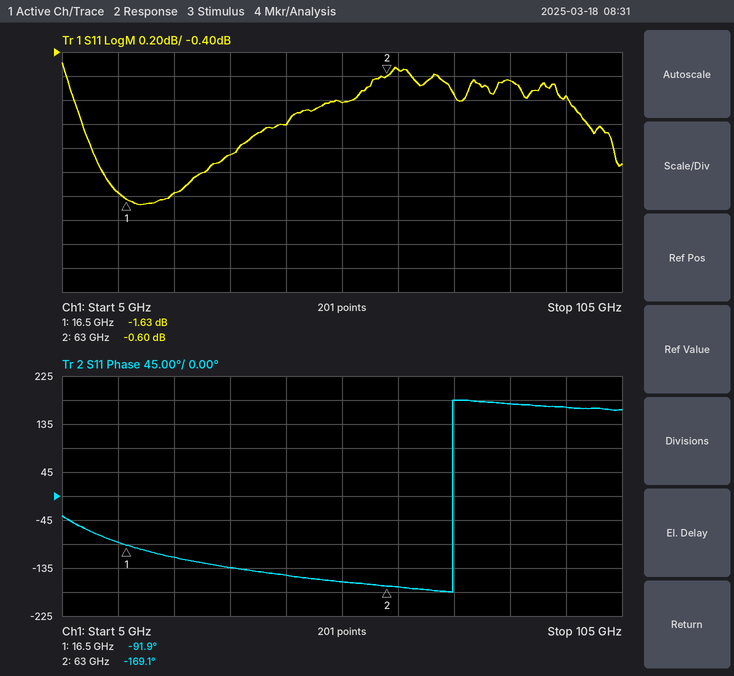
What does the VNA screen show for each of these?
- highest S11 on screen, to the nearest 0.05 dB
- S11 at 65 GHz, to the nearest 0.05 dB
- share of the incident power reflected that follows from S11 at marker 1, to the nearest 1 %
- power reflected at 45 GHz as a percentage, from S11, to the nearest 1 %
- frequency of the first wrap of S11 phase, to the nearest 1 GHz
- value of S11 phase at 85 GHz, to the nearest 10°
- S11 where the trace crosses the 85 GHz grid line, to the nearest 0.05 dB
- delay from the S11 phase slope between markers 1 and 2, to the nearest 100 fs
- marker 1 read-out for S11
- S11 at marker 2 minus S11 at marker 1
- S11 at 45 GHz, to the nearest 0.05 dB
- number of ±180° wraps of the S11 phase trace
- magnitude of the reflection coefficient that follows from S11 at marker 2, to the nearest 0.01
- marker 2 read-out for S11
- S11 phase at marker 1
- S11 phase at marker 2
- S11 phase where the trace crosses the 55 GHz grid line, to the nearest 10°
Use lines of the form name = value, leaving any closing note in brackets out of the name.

highest S11 on screen, to the nearest 0.05 dB = -0.50 dB
S11 at 65 GHz, to the nearest 0.05 dB = -0.55 dB
share of the incident power reflected that follows from S11 at marker 1, to the nearest 1 % = 69 %
power reflected at 45 GHz as a percentage, from S11, to the nearest 1 % = 79 %
frequency of the first wrap of S11 phase, to the nearest 1 GHz = 75 GHz
value of S11 phase at 85 GHz, to the nearest 10° = 170°
S11 where the trace crosses the 85 GHz grid line, to the nearest 0.05 dB = -0.65 dB
delay from the S11 phase slope between markers 1 and 2, to the nearest 100 fs = 4.6 ps
marker 1 read-out for S11 = -1.63 dB
S11 at marker 2 minus S11 at marker 1 = 1.03 dB
S11 at 45 GHz, to the nearest 0.05 dB = -1.00 dB
number of ±180° wraps of the S11 phase trace = 1
magnitude of the reflection coefficient that follows from S11 at marker 2, to the nearest 0.01 = 0.93
marker 2 read-out for S11 = -0.60 dB
S11 phase at marker 1 = -91.9°
S11 phase at marker 2 = -169.1°
S11 phase where the trace crosses the 55 GHz grid line, to the nearest 10° = -160°
